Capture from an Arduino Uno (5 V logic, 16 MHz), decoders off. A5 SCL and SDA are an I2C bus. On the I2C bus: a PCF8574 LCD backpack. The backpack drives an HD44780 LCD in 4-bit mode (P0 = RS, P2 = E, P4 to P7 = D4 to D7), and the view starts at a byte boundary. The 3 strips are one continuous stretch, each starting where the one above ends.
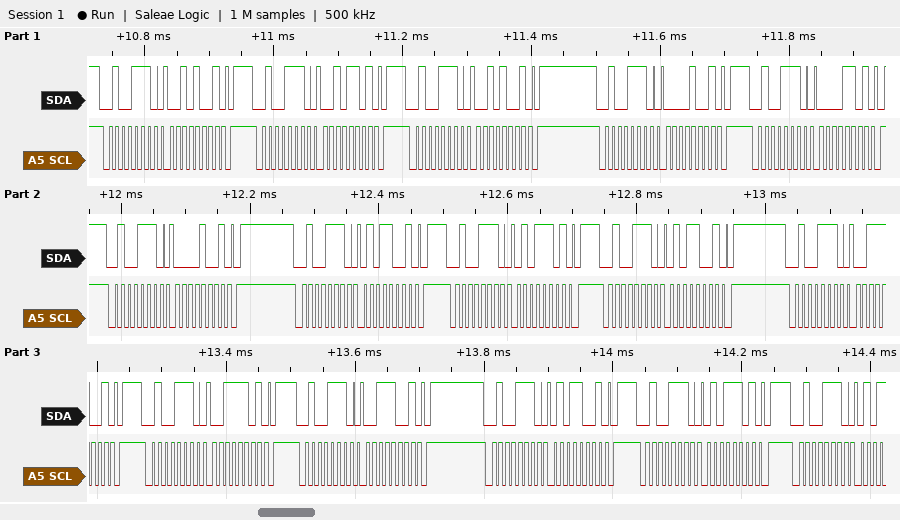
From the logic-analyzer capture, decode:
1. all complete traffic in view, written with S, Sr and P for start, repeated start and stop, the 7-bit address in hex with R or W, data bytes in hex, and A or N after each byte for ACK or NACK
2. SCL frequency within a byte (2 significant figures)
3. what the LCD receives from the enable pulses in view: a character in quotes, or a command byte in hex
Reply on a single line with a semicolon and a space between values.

S 27W A 29 A P S 27W A 2D A P S 27W A 29 A P S 27W A 09 A P S 27W A 0D A P S 27W A 09 A P S 27W A 59 A P S 27W A 5D A P S 27W A 59 A P S 27W A 39 A P S 27W A 3D A P S 27W A 39 A P S 27W A 59 A P S 27W A 5D A P S 27W A; 100 kHz; ' ' 'S'
